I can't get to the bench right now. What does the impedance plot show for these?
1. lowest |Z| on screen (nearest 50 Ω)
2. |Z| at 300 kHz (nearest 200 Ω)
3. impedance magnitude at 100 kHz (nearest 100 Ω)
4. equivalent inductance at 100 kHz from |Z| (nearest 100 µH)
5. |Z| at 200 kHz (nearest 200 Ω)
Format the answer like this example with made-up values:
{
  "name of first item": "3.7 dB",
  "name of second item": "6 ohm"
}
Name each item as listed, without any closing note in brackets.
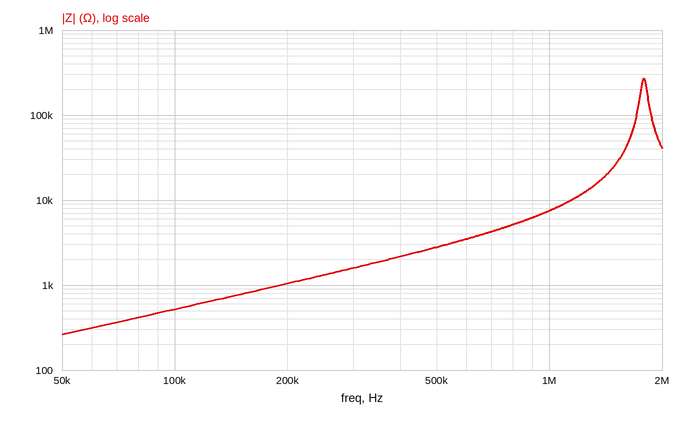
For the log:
{
  "lowest |Z| on screen": "250 Ω",
  "|Z| at 300 kHz": "1.6 kΩ",
  "impedance magnitude at 100 kHz": "500 Ω",
  "equivalent inductance at 100 kHz from |Z|": "800 µH",
  "|Z| at 200 kHz": "1.0 kΩ"
}
